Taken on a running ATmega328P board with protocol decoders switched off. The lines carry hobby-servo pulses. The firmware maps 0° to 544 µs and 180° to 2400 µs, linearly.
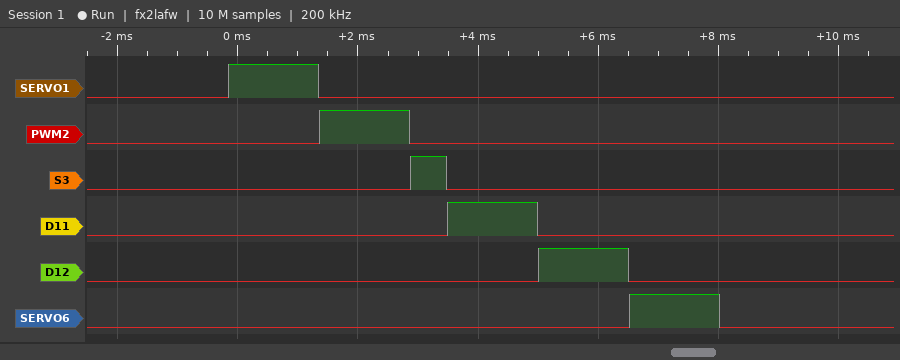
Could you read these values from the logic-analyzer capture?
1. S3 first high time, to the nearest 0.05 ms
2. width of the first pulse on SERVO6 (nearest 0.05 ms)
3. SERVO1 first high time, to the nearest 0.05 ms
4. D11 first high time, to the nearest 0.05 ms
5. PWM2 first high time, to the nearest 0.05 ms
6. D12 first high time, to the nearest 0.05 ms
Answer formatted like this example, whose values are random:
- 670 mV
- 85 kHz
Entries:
- 0.60 ms
- 1.50 ms
- 1.50 ms
- 1.50 ms
- 1.50 ms
- 1.50 ms
